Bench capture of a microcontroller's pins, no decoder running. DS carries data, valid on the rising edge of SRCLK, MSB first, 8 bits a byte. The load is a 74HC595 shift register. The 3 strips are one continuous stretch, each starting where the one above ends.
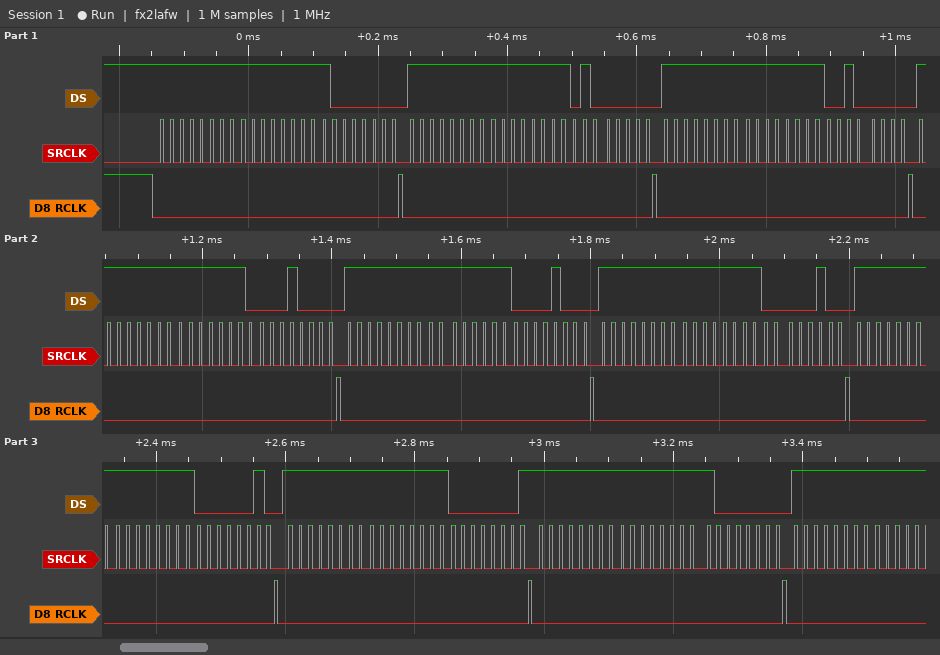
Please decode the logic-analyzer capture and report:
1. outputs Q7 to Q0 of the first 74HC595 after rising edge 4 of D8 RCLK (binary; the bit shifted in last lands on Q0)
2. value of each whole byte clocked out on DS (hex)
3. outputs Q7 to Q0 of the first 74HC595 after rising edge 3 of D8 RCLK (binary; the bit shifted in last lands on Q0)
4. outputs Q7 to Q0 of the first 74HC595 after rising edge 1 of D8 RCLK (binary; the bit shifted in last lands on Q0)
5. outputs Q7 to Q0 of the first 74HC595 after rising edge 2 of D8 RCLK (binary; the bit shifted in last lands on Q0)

00010000
FF FF 80 FF FF 40 FF FF 20 FF FE 10 FF FF 08 FF FF 04 FF FF 02 FF FF 01 FF FF 80 FF
00100000
10000000
01000000
